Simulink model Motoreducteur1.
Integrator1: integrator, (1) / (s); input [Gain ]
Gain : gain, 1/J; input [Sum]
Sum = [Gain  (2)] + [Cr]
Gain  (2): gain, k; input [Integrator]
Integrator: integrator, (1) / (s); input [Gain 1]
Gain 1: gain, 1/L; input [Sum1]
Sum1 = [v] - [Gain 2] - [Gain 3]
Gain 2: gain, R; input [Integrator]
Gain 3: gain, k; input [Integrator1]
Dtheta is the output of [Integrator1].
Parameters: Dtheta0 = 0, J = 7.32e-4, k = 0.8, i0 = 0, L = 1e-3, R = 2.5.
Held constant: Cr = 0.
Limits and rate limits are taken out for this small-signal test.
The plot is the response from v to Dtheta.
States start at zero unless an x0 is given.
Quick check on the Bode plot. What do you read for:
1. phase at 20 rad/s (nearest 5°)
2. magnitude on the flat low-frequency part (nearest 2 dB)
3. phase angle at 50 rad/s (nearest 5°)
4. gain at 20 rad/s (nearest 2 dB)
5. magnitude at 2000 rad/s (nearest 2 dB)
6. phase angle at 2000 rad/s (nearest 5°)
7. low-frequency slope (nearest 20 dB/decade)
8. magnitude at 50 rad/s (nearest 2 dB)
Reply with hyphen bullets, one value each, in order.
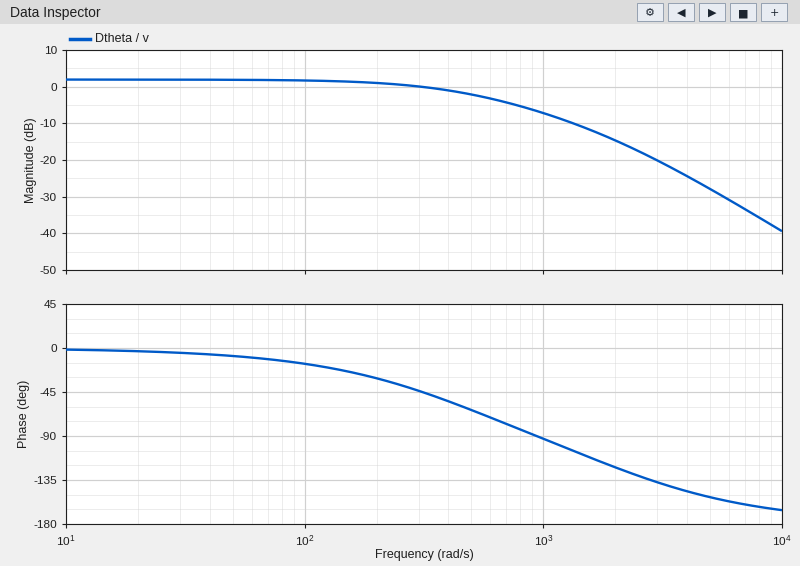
- -5°
- 2 dB
- -10°
- 2 dB
- -14 dB
- -120°
- 0 dB/decade
- 2 dB
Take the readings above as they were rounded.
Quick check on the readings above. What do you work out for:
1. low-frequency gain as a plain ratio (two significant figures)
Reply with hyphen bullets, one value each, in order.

- 1.3
